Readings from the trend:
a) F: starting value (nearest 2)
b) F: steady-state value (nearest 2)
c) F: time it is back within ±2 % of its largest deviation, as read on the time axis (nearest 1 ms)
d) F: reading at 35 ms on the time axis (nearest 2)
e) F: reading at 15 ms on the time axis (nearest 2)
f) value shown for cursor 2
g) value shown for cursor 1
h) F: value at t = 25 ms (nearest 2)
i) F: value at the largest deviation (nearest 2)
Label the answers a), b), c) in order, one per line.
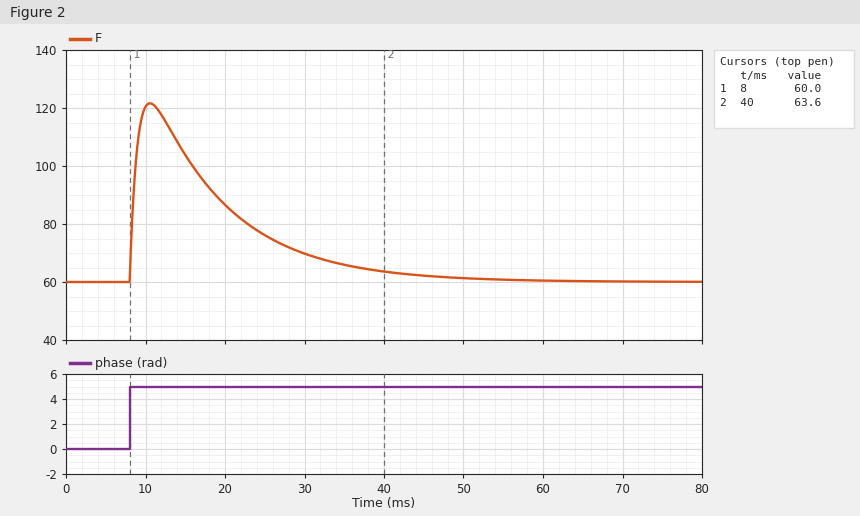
a) 60
b) 60
c) 51 ms
d) 66
e) 104
f) 63.6
g) 60.0
h) 76
i) 122
